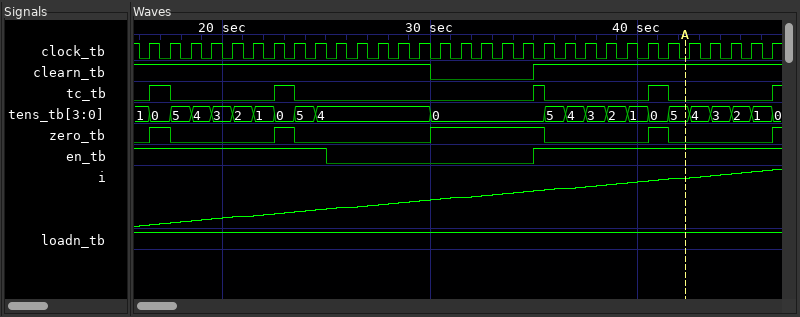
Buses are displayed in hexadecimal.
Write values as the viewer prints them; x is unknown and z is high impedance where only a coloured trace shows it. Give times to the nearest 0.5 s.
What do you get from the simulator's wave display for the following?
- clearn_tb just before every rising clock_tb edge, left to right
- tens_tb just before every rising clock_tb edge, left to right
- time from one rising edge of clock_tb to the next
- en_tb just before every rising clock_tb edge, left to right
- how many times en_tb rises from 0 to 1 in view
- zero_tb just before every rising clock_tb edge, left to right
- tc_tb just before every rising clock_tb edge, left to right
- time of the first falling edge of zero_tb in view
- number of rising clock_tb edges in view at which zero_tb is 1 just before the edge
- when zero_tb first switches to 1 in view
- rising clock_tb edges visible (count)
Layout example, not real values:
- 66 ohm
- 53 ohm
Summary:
- 1 1 1 1 1 1 1 1 1 1 1 1 1 1 0 0 0 0 0 1 1 1 1 1 1 1 1 1 1 1 1
- 1, 0, 5, 4, 3, 2, 1, 0, 5, 4, 4, 4, 4, 4, 0, 0, 0, 0, 0, 0, 5, 4, 3, 2, 1, 0, 5, 4, 3, 2, 1
- 1 s
- 1 1 1 1 1 1 1 1 1 0 0 0 0 0 0 0 0 0 0 1 1 1 1 1 1 1 1 1 1 1 1
- 1
- 0 1 0 0 0 0 0 1 0 0 0 0 0 0 1 1 1 1 1 1 0 0 0 0 0 1 0 0 0 0 0
- 0 1 0 0 0 0 0 1 0 0 0 0 0 0 0 0 0 0 0 1 0 0 0 0 0 1 0 0 0 0 0
- 17.5 s
- 9
- 16.5 s
- 31
